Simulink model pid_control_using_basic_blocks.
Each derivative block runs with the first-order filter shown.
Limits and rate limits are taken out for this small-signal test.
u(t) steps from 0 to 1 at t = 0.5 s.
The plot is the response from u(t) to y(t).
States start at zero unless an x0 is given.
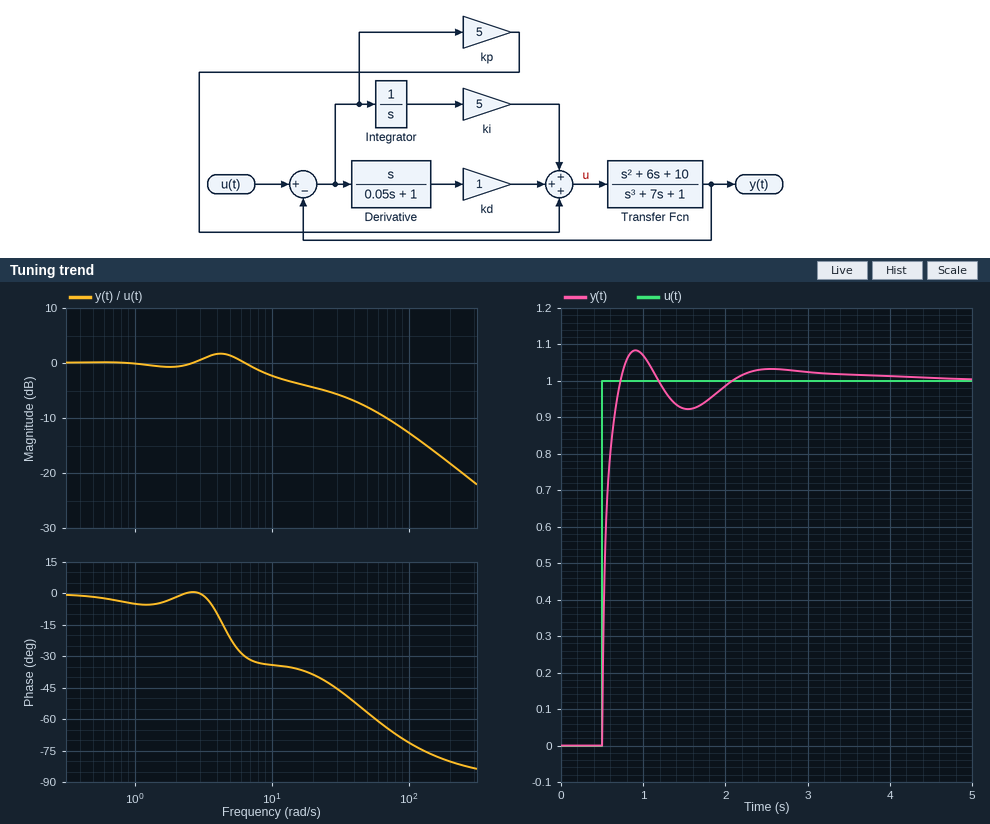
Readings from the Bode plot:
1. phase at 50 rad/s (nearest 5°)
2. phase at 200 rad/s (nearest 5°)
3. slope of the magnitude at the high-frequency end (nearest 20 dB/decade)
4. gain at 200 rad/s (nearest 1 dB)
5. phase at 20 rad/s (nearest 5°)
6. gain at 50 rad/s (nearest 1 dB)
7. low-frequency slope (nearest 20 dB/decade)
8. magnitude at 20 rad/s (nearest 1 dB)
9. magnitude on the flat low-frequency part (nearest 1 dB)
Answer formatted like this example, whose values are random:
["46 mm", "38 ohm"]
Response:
["-55°", "-80°", "-20 dB/decade", "-18 dB", "-40°", "-8 dB", "0 dB/decade", "-4 dB", "0 dB"]
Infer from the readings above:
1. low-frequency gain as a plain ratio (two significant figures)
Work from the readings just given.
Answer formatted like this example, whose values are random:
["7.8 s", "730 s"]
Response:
["1.0"]
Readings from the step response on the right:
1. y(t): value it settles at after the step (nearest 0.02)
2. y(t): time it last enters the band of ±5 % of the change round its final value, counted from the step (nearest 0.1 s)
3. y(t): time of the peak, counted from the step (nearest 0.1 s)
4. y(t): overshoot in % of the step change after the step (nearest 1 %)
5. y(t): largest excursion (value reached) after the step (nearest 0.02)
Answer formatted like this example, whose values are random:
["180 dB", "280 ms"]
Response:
["1.00", "1.3 s", "0.4 s", "8 %", "1.08"]
